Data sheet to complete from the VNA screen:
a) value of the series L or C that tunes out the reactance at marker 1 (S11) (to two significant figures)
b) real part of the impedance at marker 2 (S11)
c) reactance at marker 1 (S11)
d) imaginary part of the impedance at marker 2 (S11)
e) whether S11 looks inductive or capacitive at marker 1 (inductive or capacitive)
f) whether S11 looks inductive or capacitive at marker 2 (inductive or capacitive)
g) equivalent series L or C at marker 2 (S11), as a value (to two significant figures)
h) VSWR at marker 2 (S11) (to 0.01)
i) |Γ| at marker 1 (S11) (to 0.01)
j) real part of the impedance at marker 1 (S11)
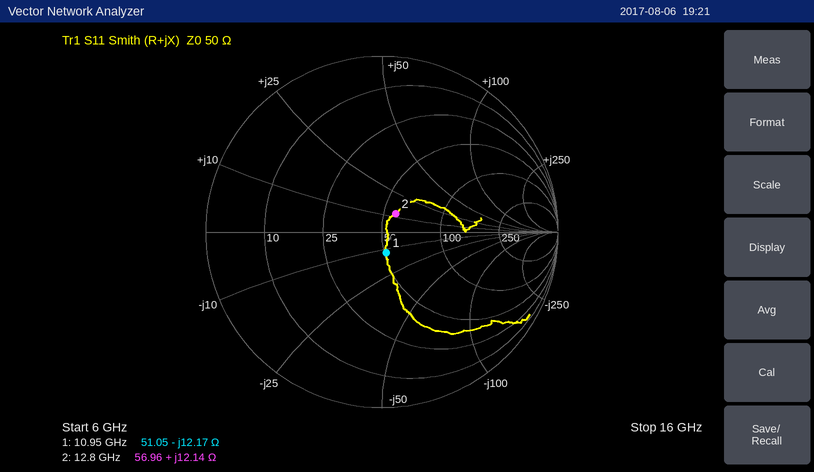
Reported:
180 pH
56.96 Ω
-12.17 Ω
+12.14 Ω
capacitive
inductive
150 pH
1.30
0.12
51.05 Ω
